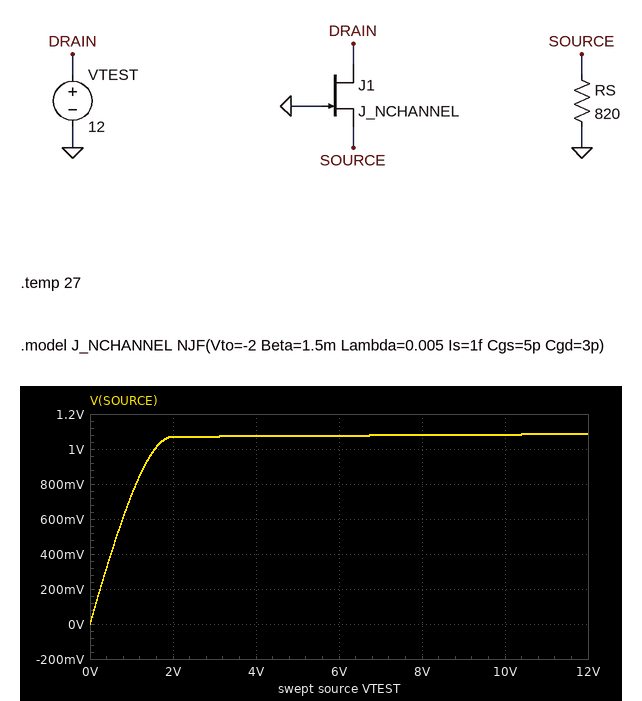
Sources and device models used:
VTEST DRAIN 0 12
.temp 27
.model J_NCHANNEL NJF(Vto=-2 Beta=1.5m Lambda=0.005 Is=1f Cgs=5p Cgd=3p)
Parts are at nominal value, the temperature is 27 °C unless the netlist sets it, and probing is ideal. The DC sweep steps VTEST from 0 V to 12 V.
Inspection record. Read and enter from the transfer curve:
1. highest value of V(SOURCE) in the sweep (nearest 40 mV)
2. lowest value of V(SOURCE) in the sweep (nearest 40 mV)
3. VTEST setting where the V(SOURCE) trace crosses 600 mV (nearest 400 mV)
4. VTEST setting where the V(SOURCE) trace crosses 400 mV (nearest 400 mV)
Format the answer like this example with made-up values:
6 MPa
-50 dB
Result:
1.08 V
0 V
800 mV
400 mV
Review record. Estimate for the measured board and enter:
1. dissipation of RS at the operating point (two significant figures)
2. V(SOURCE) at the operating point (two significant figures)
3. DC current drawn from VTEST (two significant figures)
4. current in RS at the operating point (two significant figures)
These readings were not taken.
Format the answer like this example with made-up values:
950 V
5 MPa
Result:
1.4 mW
1.1 V
1.3 mA
1.3 mA
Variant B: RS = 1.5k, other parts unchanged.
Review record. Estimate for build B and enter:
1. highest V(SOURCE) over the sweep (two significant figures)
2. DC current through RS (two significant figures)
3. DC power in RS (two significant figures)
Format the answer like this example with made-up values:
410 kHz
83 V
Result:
1.3 V
850 µA
1.1 mW
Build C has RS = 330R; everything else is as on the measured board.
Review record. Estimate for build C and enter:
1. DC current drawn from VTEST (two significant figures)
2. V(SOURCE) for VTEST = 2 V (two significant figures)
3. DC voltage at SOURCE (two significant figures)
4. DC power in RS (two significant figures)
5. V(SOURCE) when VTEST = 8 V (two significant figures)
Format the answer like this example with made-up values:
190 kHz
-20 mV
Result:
2.4 mA
760 mV
780 mV
1.8 mW
770 mV
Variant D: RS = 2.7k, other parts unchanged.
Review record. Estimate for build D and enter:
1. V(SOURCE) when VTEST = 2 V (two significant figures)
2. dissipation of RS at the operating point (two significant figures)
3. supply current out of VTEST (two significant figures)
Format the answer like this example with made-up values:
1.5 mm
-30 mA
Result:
1.4 V
750 µW
530 µA
